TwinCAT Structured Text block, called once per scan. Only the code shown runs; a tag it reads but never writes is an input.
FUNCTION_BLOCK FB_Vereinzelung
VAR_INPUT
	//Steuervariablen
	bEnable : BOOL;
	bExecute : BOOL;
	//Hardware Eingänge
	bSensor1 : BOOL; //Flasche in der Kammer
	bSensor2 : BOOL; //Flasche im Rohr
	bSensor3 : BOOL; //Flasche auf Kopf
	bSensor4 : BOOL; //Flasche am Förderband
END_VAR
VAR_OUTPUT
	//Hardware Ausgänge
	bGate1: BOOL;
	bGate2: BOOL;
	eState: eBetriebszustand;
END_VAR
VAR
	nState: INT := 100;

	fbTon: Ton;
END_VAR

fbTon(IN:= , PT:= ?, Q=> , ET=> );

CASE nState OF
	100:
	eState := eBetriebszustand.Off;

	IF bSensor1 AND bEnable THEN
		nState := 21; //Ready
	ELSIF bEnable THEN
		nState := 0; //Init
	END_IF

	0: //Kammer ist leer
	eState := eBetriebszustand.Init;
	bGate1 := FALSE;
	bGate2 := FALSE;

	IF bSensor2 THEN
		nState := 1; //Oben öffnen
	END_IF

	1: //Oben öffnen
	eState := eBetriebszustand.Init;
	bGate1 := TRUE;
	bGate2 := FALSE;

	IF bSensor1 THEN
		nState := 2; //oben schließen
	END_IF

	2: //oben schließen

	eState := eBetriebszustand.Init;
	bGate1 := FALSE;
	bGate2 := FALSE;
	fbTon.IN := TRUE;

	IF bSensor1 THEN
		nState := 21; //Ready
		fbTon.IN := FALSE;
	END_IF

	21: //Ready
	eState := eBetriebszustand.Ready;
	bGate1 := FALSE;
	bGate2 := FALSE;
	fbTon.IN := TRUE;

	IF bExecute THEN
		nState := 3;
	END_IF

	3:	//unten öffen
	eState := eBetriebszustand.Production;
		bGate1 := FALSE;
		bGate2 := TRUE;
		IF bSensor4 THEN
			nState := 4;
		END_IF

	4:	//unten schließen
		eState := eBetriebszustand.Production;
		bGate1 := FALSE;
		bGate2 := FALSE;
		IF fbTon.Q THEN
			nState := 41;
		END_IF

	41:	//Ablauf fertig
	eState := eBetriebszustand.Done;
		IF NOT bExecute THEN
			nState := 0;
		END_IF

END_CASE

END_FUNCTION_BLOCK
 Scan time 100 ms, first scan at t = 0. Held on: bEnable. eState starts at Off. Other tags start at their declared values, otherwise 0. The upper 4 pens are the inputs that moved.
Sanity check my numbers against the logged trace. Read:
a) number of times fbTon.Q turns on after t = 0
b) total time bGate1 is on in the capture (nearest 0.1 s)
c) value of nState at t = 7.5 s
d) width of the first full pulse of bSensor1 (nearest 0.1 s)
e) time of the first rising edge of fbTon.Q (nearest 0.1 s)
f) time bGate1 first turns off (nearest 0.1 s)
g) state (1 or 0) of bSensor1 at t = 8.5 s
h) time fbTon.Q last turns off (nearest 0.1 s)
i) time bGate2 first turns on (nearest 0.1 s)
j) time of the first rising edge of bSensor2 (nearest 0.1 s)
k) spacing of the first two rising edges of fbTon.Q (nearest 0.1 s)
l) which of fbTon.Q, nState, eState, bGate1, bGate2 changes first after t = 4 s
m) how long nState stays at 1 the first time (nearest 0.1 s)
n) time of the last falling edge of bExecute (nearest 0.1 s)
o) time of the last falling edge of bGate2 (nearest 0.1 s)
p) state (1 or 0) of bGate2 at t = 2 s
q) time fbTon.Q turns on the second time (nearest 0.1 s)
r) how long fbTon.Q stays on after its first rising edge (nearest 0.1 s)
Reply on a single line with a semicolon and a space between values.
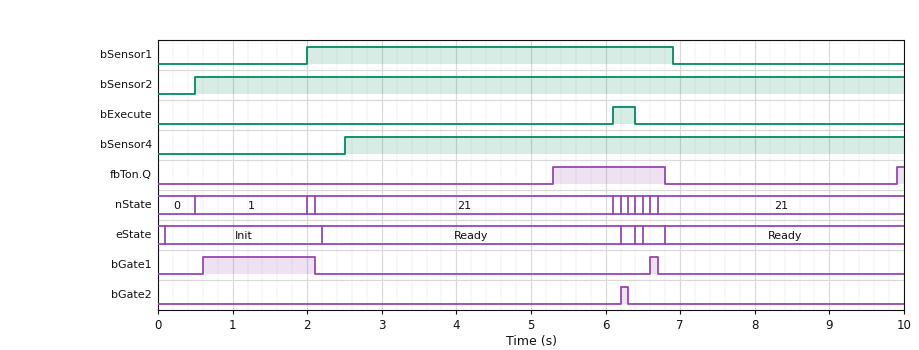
2; 1.6 s; 21; 4.9 s; 5.3 s; 2.1 s; 0; 6.8 s; 6.2 s; 0.5 s; 4.6 s; fbTon.Q; 1.5 s; 6.4 s; 6.3 s; 0; 9.9 s; 1.5 s
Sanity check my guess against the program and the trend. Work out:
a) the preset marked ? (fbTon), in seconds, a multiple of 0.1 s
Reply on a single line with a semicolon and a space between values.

3.0 s
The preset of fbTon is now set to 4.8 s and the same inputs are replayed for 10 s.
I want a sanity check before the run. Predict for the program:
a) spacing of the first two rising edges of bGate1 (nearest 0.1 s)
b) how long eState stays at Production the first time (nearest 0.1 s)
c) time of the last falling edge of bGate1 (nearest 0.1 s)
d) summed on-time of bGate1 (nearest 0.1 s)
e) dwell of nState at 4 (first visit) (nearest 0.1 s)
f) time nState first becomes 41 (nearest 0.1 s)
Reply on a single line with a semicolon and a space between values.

6.8 s; 1.0 s; 2.1 s; 4.1 s; 0.9 s; 7.1 s
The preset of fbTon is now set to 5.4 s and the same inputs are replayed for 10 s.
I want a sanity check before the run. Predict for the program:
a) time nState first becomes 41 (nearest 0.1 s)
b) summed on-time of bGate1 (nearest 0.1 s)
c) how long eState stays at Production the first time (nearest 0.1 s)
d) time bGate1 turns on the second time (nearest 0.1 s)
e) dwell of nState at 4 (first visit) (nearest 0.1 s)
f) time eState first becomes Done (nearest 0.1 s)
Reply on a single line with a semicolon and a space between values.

7.7 s; 3.5 s; 1.6 s; 8.0 s; 1.5 s; 7.8 s
